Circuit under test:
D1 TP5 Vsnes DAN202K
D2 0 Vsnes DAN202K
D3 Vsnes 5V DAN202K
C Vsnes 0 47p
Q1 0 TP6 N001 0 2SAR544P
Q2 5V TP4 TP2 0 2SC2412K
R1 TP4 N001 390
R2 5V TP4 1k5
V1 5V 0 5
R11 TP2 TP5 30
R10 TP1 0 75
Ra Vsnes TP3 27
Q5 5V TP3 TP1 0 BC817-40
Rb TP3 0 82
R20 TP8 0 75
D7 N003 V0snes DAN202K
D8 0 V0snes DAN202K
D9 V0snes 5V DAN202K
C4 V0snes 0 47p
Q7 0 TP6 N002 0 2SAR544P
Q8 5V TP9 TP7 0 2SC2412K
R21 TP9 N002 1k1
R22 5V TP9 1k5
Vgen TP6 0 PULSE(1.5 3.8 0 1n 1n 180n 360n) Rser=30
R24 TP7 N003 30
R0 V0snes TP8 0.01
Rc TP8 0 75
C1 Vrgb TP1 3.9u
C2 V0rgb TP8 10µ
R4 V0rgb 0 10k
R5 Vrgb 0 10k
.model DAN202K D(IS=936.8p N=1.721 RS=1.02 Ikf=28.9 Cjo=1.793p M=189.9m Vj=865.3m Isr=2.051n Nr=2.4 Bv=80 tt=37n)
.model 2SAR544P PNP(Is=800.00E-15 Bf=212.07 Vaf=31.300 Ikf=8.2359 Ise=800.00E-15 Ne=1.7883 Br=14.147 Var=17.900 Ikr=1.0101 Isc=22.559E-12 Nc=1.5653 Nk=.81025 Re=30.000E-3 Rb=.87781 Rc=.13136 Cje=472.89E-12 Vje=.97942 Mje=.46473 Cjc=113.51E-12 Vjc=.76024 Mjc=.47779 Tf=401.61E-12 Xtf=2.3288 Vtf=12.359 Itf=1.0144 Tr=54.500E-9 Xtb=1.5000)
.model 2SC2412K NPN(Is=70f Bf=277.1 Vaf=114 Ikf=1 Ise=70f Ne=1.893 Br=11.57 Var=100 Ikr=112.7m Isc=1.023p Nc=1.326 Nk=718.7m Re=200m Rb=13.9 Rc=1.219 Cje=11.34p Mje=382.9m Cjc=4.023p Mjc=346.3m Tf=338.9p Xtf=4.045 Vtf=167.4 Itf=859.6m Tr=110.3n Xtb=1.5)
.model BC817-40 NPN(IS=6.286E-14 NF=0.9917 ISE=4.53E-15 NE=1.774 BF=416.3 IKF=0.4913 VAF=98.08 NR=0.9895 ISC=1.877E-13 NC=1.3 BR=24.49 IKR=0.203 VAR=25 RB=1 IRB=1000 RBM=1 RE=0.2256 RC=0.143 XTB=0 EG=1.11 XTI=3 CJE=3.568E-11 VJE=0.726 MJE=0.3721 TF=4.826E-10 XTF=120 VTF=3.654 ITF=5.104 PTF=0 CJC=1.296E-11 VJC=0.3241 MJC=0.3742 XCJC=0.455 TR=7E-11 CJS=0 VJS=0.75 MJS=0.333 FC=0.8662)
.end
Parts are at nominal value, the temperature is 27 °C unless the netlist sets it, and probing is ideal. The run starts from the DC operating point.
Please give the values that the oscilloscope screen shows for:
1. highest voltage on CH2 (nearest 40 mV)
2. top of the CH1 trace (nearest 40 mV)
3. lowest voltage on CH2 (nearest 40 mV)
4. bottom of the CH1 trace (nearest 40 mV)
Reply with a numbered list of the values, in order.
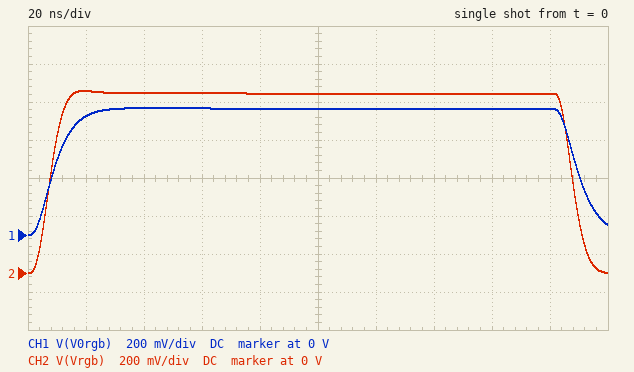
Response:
1. 960 mV
2. 680 mV
3. 0 V
4. 0 V
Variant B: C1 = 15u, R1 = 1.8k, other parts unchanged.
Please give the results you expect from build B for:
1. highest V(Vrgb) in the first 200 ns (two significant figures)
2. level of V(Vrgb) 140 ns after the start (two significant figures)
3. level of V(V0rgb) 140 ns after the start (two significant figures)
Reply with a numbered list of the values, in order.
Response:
1. 560 mV
2. 550 mV
3. 660 mV
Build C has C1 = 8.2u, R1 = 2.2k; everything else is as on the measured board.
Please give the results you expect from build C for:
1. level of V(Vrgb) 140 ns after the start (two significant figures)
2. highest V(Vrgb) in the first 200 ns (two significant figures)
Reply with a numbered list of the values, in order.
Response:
1. 490 mV
2. 500 mV
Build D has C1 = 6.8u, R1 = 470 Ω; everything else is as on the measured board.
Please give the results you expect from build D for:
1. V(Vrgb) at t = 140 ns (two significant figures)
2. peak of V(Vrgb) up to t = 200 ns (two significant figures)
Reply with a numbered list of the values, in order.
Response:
1. 910 mV
2. 930 mV
